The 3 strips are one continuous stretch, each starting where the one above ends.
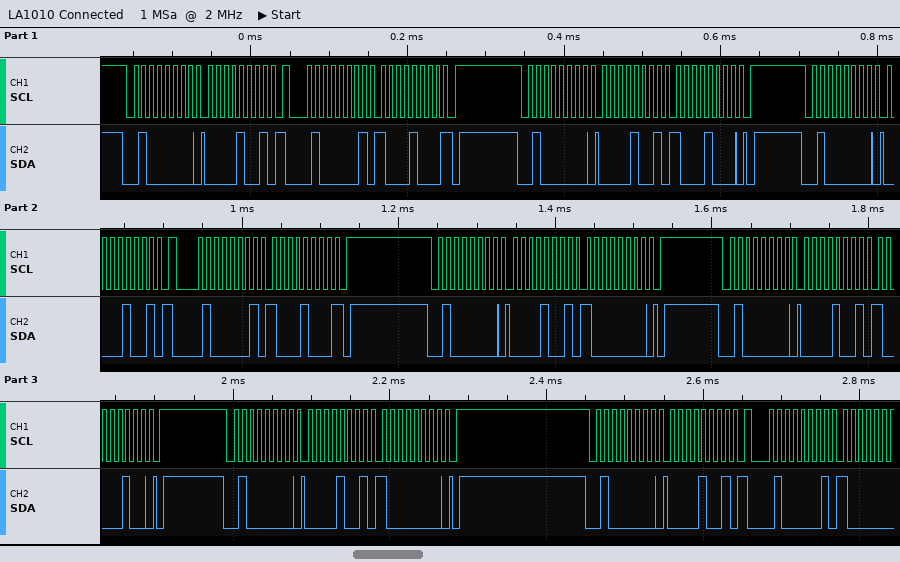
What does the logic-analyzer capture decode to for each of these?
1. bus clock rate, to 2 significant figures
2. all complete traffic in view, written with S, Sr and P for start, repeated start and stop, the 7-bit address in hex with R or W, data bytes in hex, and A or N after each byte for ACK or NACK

100 kHz
S 20W A 09 A Sr 20R A 88 N P S 20W A 09 A 88 A P S 20W A 09 A Sr 20R A 88 N P S 20W A 09 A 80 A P S 20W A 09 A 84 A P S 20W A 09 A 80 A P S 20W A 09 A Sr 20R A
